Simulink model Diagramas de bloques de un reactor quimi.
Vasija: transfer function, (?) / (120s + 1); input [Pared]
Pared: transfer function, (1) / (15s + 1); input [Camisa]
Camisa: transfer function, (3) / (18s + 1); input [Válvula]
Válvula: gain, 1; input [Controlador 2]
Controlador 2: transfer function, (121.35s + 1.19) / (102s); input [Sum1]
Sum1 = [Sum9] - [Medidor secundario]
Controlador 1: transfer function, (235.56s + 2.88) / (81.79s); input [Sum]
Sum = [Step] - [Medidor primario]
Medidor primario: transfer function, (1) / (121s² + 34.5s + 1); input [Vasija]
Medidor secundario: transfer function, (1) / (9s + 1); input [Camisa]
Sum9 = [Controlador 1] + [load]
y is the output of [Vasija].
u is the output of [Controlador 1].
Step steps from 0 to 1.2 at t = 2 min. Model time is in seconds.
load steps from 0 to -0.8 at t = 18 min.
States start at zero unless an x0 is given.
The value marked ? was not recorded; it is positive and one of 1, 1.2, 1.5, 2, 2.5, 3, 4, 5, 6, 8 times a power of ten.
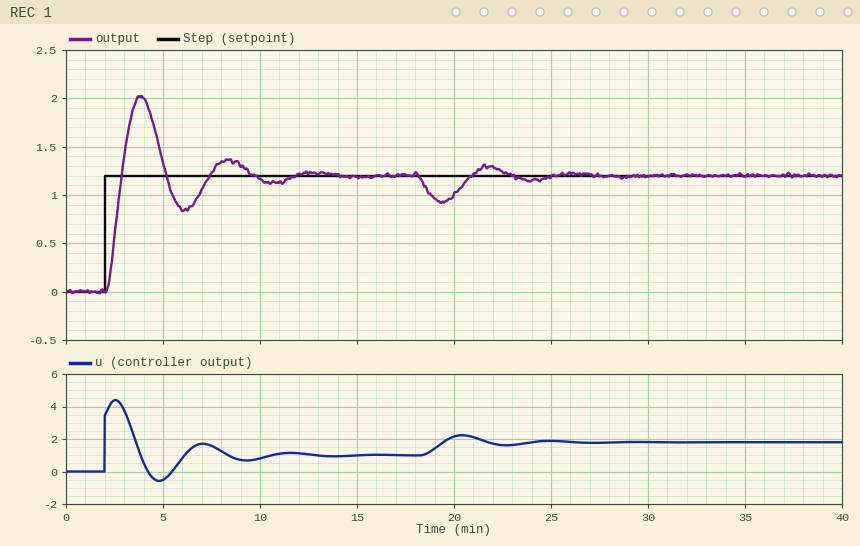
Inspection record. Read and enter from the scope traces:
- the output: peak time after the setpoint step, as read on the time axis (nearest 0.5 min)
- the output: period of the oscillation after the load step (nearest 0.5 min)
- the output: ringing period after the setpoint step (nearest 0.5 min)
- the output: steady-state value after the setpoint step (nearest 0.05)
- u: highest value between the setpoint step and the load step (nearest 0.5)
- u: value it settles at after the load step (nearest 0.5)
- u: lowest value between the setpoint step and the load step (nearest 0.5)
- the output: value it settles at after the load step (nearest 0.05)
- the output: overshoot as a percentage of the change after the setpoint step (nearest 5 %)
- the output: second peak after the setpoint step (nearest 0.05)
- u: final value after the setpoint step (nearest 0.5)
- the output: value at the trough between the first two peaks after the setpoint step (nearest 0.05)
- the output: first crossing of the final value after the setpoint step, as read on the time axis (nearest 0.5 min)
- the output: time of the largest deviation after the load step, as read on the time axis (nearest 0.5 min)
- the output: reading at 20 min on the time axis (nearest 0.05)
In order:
4.0 min
4.5 min
4.5 min
1.20
4.5
2.0
-0.5
1.20
70 %
1.35
1.0
0.85
3.0 min
19.5 min
1.00
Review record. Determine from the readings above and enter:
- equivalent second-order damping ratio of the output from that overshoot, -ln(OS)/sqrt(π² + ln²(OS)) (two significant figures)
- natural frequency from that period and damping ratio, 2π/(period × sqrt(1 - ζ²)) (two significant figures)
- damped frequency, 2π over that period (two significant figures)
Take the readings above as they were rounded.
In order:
0.11
1.4 rad/min
1.4 rad/min
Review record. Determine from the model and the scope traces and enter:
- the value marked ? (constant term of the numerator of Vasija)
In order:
1.2
